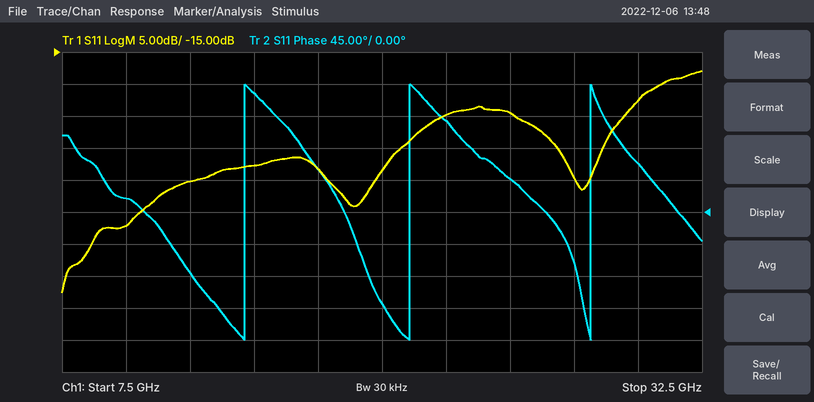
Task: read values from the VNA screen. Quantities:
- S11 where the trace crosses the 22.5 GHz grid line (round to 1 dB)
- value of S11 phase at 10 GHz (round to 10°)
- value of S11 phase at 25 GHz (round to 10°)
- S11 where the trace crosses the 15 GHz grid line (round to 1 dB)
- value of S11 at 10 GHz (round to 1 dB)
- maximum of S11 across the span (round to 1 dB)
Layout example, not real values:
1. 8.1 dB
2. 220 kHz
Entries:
1. -25 dB
2. 20°
3. 50°
4. -33 dB
5. -42 dB
6. -18 dB
